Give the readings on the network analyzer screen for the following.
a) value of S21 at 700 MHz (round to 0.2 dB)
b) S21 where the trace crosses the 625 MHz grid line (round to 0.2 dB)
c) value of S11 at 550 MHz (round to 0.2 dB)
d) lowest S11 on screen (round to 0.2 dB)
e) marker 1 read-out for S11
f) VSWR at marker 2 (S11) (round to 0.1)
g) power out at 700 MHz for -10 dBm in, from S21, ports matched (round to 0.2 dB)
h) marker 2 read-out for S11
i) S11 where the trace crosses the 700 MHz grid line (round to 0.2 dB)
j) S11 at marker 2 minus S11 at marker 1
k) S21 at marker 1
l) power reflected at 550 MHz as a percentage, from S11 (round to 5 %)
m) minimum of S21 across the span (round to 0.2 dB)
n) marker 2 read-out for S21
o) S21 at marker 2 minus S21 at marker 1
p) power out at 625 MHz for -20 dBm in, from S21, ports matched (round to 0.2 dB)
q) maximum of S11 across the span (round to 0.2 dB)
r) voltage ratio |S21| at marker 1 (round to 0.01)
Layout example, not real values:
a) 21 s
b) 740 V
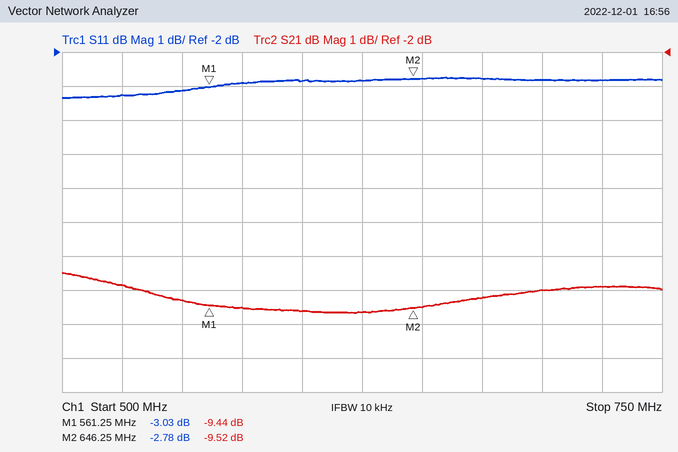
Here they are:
a) -9.0 dB
b) -9.6 dB
c) -3.2 dB
d) -3.4 dB
e) -3.03 dB
f) 6.3
g) -19.0 dBm
h) -2.78 dB
i) -2.8 dB
j) 0.25 dB
k) -9.44 dB
l) 50 %
m) -9.6 dB
n) -9.52 dB
o) -0.08 dB
p) -29.6 dBm
q) -2.8 dB
r) 0.34
